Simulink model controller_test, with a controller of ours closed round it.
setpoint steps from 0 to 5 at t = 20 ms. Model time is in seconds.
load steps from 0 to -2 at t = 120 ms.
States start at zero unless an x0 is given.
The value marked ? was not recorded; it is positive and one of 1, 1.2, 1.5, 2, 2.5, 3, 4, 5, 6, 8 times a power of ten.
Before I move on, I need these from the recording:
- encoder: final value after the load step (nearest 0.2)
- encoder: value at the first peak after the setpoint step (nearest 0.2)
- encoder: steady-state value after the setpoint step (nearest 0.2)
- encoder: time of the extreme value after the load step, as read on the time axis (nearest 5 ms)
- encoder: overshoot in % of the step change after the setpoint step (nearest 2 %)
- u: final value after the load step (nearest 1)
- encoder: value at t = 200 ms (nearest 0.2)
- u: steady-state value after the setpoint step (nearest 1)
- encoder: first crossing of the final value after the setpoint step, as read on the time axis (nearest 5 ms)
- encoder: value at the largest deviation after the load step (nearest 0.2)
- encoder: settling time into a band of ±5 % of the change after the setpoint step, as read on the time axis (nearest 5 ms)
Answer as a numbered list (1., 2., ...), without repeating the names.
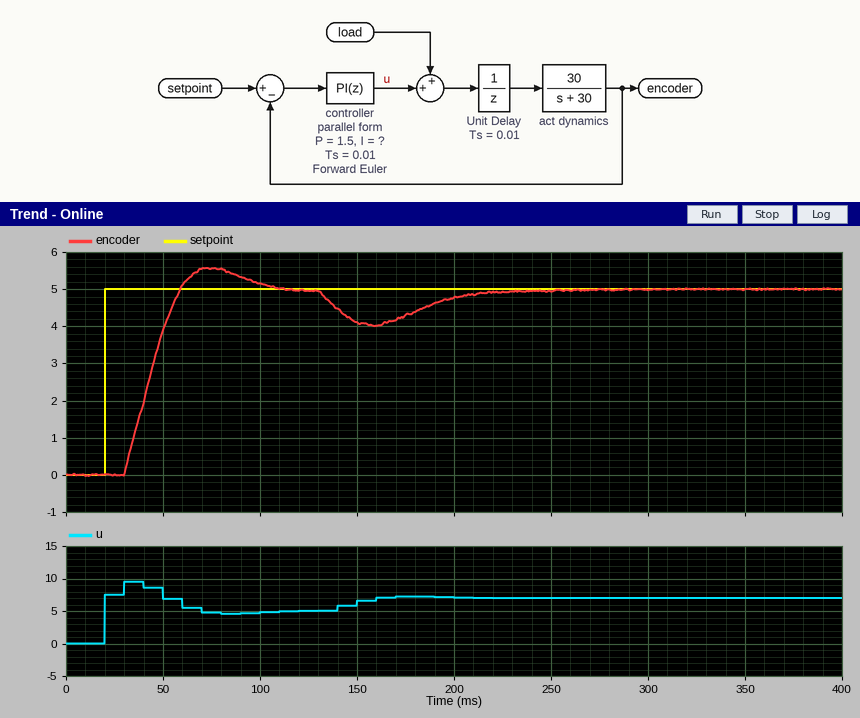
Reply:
1. 5.0
2. 5.6
3. 5.0
4. 160 ms
5. 12 %
6. 7
7. 4.8
8. 5
9. 60 ms
10. 4.0
11. 95 ms
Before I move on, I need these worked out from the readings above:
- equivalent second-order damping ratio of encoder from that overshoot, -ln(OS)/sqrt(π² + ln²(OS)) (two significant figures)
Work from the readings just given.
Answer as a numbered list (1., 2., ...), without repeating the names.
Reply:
1. 0.56
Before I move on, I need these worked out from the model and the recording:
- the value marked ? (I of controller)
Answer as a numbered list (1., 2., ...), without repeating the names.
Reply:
1. 40
